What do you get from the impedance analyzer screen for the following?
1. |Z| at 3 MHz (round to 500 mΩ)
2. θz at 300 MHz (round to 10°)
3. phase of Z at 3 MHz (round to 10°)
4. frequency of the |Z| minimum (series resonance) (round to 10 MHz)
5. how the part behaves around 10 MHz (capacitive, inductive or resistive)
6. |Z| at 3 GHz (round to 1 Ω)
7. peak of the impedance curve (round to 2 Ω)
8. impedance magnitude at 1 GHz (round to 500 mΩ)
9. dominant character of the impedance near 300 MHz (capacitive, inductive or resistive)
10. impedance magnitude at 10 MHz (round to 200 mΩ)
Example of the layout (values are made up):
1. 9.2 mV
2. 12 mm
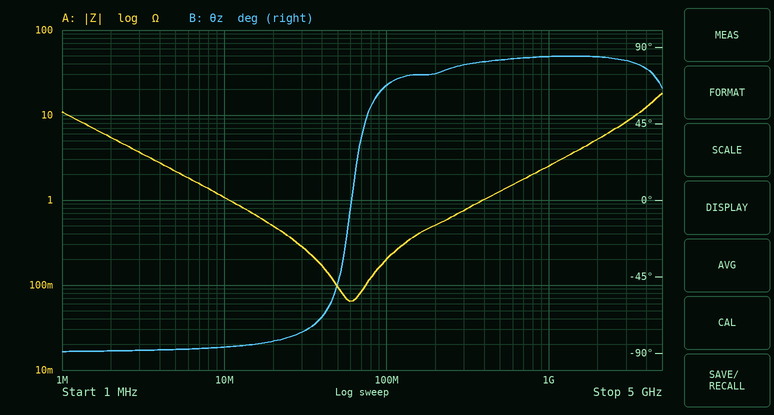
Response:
1. 3.5 Ω
2. 80°
3. -90°
4. 60 MHz
5. capacitive
6. 8 Ω
7. 18 Ω
8. 2.5 Ω
9. inductive
10. 1.0 Ω
